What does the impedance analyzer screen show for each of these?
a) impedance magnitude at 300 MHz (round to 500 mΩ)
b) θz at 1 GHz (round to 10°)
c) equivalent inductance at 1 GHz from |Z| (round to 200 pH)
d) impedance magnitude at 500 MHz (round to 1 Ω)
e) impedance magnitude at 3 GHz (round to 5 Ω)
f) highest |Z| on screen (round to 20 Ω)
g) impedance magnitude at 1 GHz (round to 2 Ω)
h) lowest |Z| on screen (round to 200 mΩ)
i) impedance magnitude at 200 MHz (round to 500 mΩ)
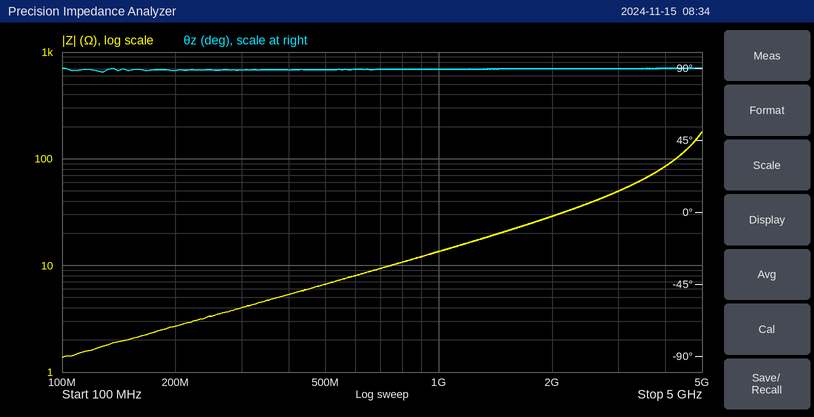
4.0 Ω
90°
2.2 nH
7 Ω
50 Ω
180 Ω
14 Ω
1.4 Ω
2.5 Ω
